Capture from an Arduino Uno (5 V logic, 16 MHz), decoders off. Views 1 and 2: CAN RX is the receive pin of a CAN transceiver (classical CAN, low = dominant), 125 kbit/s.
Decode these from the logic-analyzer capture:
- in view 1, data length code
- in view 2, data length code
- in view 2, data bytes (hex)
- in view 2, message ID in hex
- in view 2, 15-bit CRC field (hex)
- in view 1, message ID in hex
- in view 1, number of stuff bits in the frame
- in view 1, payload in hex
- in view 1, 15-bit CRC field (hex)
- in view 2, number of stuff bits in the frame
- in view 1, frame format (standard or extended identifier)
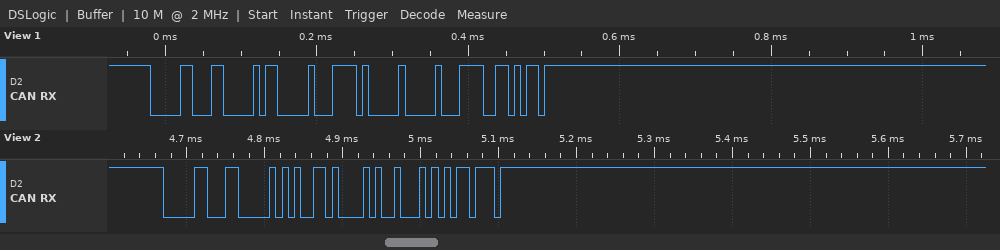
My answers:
3
2
9A 14
0x046
0x455B
0x046
5
00 F4 00
0x0F35
2
standard
